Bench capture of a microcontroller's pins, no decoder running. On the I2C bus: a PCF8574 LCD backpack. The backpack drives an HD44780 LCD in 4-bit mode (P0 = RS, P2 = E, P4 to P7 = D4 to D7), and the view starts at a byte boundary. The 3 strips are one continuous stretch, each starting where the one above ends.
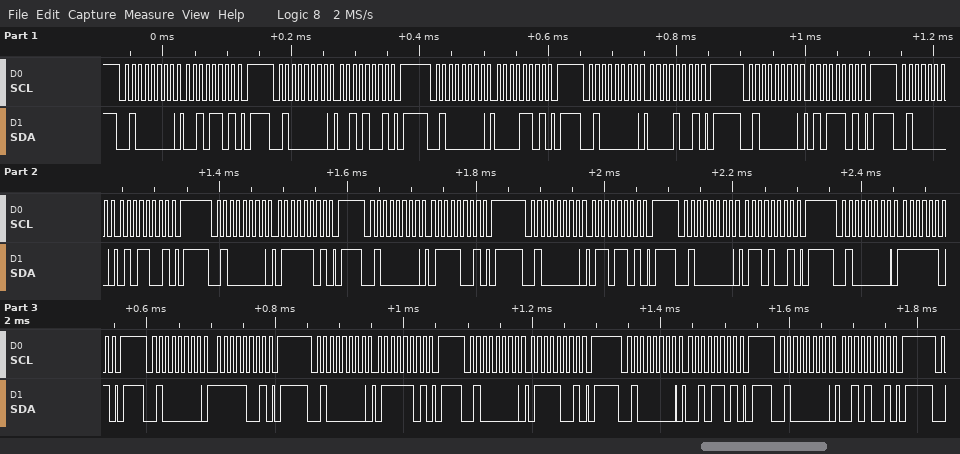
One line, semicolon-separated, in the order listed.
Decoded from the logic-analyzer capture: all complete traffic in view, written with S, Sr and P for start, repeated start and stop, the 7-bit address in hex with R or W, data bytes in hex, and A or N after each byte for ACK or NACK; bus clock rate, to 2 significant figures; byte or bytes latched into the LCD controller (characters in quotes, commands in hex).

S 20W A 2D A P S 20W A 29 A P S 20W A 0D A P S 20W A 09 A P S 20W A 5D A P S 20W A 59 A P S 20W A 7D A P S 20W A 79 A P S 20W A 6D A P S 20W A 69 A P S 20W A FD A P S 20W A F9 A P S 20W A 7D A P S 20W A 79 A P S 20W A 2D A P S 20W A 29 A P; 100 kHz; ' ' 'W' 'o' 'r'
